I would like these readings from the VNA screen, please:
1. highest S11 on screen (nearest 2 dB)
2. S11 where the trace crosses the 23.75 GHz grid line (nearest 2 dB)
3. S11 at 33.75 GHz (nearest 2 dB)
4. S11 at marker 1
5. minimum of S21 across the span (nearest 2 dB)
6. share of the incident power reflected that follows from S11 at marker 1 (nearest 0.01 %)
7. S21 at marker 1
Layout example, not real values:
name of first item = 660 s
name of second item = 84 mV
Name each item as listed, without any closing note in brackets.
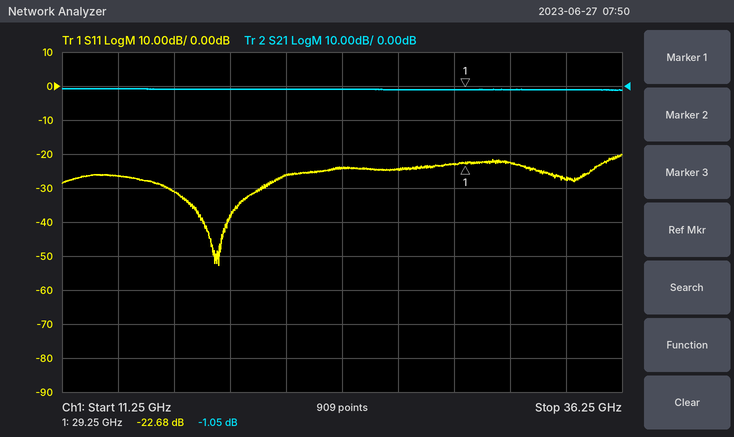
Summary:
highest S11 on screen = -20 dB
S11 where the trace crosses the 23.75 GHz grid line = -24 dB
S11 at 33.75 GHz = -28 dB
S11 at marker 1 = -22.68 dB
minimum of S21 across the span = -2 dB
share of the incident power reflected that follows from S11 at marker 1 = 0.54 %
S21 at marker 1 = -1.05 dB
